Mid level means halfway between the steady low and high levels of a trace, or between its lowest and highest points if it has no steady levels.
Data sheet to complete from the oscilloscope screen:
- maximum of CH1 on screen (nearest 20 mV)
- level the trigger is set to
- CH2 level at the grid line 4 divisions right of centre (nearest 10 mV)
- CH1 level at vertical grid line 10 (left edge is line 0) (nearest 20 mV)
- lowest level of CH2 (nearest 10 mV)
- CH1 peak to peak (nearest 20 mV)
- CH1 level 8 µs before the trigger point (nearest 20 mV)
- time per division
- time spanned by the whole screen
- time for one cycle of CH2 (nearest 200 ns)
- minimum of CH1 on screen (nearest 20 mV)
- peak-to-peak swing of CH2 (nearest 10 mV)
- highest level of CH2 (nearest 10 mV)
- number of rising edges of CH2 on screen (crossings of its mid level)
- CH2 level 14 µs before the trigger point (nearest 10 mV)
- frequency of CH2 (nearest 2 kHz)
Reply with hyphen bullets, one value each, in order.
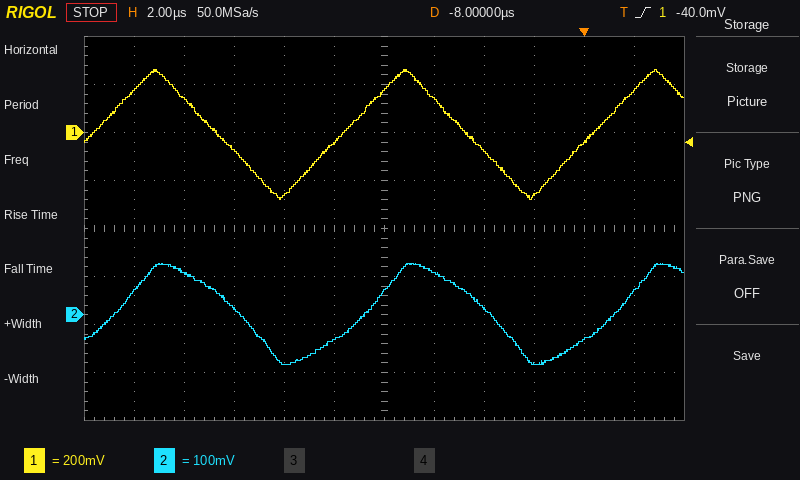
- 260 mV
- -40.0 mV
- -50 mV
- -40 mV
- -100 mV
- 540 mV
- 180 mV
- 2 µs
- 24 µs
- 10.0 µs
- -280 mV
- 210 mV
- 110 mV
- 3
- 10 mV
- 100 kHz
